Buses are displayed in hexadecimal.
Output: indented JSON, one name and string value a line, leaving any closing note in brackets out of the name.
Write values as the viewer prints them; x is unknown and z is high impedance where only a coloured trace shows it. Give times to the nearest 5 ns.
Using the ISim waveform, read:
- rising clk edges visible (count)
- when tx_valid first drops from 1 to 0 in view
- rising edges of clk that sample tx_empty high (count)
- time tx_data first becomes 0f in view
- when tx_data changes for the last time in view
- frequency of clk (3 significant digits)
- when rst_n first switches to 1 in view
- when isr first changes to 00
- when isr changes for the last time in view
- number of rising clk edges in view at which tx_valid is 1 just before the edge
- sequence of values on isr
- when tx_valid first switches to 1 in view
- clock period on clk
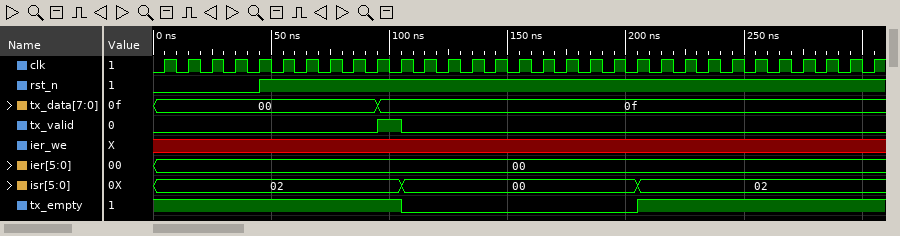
{
  "rising clk edges visible": "31",
  "when tx_valid first drops from 1 to 0 in view": "105 ns",
  "rising edges of clk that sample tx_empty high": "21",
  "time tx_data first becomes 0f in view": "95 ns",
  "when tx_data changes for the last time in view": "95 ns",
  "frequency of clk": "100 MHz",
  "when rst_n first switches to 1 in view": "45 ns",
  "when isr first changes to 00": "105 ns",
  "when isr changes for the last time in view": "205 ns",
  "number of rising clk edges in view at which tx_valid is 1 just before the edge": "1",
  "sequence of values on isr": "02, 00, 02",
  "when tx_valid first switches to 1 in view": "95 ns",
  "clock period on clk": "10 ns"
}
